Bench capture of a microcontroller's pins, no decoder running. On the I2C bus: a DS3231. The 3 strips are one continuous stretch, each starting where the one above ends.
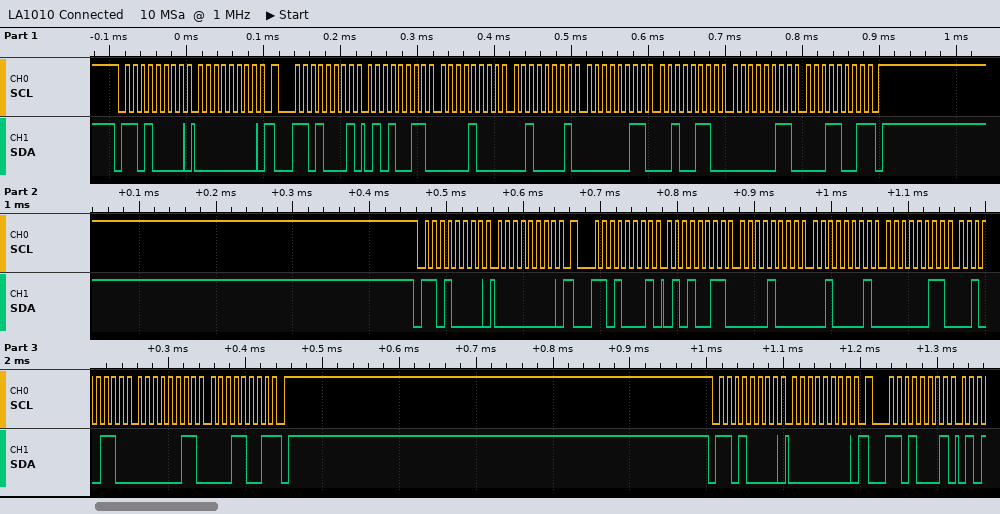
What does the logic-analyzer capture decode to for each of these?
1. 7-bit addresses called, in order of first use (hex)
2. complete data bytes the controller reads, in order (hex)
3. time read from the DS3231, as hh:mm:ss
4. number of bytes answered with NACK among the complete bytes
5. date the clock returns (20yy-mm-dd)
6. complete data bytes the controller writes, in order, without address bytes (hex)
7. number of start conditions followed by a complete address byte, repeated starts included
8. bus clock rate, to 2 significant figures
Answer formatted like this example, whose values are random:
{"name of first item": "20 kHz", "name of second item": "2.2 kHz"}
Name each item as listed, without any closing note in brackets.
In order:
{"7-bit addresses called, in order of first use": "0x68", "complete data bytes the controller reads, in order": "53 08 21 03 26 03 19 53 08 21 03 26 03 19", "time read from the DS3231, as hh:mm:ss": "21:08:53", "number of bytes answered with NACK among the complete bytes": "2", "date the clock returns": "2019-03-26", "complete data bytes the controller writes, in order, without address bytes": "00 00 00", "number of start conditions followed by a complete address byte, repeated starts included": "6", "bus clock rate, to 2 significant figures": "100 kHz"}
